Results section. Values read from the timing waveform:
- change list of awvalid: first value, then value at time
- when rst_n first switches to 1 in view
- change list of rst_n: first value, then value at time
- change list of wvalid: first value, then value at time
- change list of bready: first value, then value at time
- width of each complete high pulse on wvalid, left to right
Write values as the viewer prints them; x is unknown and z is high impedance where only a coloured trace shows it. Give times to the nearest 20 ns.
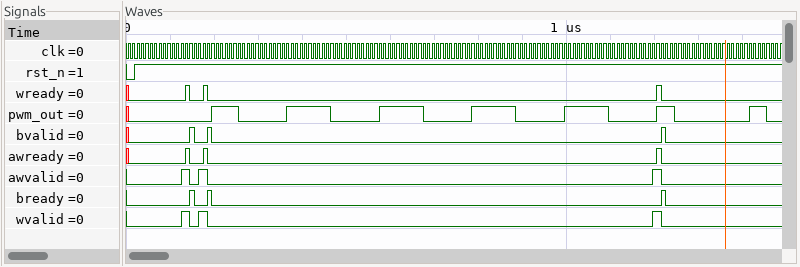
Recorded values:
0, 1 at 120 ns, 0 at 140 ns, 1 at 160 ns, 0 at 180 ns, 1 at 1200 ns, 0 at 1220 ns
20 ns
0, 1 at 20 ns
0, 1 at 120 ns, 0 at 140 ns, 1 at 160 ns, 0 at 180 ns, 1 at 1200 ns, 0 at 1220 ns
0, 1 at 140 ns, 0 at 160 ns, 1 at 180 ns, 0 at 200 ns, 1 at 1220 ns, 0 at 1220 ns
20 ns, 20 ns, 20 ns
